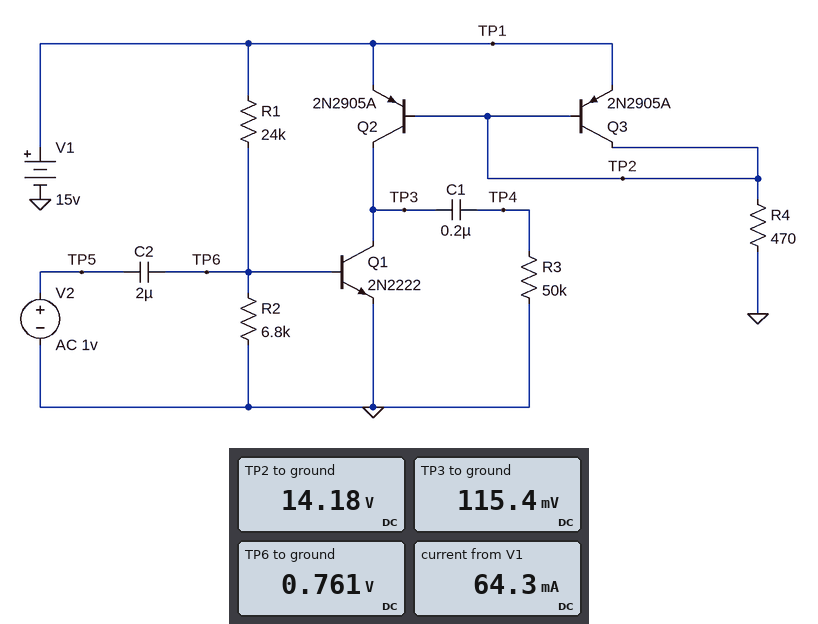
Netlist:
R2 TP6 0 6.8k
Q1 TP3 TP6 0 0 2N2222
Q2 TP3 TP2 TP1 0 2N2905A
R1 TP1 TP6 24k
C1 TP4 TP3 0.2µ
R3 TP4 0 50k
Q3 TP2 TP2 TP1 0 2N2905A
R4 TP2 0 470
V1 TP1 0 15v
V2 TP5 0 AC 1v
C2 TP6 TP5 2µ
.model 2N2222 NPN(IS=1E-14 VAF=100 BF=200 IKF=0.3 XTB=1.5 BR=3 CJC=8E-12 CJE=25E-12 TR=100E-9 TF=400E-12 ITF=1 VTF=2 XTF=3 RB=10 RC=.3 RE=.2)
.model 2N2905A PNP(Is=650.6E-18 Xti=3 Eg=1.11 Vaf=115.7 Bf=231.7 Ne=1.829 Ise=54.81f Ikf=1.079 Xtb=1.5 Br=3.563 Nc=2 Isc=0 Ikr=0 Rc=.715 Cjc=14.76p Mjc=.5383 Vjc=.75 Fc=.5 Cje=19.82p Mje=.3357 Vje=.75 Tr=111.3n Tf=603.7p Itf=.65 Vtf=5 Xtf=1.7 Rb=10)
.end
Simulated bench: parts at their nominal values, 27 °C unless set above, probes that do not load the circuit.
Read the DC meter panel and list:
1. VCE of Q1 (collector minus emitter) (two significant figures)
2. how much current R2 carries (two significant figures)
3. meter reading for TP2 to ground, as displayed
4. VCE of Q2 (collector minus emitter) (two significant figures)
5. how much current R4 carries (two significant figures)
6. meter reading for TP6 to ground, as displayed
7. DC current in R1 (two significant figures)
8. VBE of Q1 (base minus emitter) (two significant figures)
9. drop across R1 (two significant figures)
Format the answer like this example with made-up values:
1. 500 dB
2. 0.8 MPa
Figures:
1. 120 mV
2. 110 µA
3. 14.18 V
4. -15 V
5. 30 mA
6. 0.761 V
7. 590 µA
8. 760 mV
9. 14 V
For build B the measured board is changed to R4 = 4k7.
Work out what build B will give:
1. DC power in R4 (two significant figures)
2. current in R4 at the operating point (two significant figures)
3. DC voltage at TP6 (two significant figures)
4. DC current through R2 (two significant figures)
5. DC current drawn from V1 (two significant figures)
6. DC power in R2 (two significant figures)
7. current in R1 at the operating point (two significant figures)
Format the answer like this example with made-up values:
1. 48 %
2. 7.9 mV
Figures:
1. 43 mW
2. 3.0 mA
3. 700 mV
4. 100 µA
5. 7.0 mA
6. 73 µW
7. 600 µA
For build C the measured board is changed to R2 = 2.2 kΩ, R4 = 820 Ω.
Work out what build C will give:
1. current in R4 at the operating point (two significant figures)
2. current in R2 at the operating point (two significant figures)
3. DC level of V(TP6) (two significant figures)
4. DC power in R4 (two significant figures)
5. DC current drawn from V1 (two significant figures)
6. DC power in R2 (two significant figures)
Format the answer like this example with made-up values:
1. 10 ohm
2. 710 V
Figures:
1. 17 mA
2. 340 µA
3. 740 mV
4. 250 mW
5. 37 mA
6. 250 µW
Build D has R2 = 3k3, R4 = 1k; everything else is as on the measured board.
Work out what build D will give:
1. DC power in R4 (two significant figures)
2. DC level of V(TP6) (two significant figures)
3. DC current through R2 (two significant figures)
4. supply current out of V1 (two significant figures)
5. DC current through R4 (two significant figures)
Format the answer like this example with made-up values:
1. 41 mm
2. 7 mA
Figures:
1. 200 mW
2. 740 mV
3. 220 µA
4. 31 mA
5. 14 mA
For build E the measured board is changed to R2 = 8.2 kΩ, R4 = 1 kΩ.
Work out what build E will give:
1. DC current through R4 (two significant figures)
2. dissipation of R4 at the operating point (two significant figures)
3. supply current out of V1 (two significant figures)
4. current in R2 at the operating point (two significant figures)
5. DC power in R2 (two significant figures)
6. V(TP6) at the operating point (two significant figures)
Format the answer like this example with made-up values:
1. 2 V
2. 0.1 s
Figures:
1. 14 mA
2. 200 mW
3. 31 mA
4. 90 µA
5. 67 µW
6. 740 mV
